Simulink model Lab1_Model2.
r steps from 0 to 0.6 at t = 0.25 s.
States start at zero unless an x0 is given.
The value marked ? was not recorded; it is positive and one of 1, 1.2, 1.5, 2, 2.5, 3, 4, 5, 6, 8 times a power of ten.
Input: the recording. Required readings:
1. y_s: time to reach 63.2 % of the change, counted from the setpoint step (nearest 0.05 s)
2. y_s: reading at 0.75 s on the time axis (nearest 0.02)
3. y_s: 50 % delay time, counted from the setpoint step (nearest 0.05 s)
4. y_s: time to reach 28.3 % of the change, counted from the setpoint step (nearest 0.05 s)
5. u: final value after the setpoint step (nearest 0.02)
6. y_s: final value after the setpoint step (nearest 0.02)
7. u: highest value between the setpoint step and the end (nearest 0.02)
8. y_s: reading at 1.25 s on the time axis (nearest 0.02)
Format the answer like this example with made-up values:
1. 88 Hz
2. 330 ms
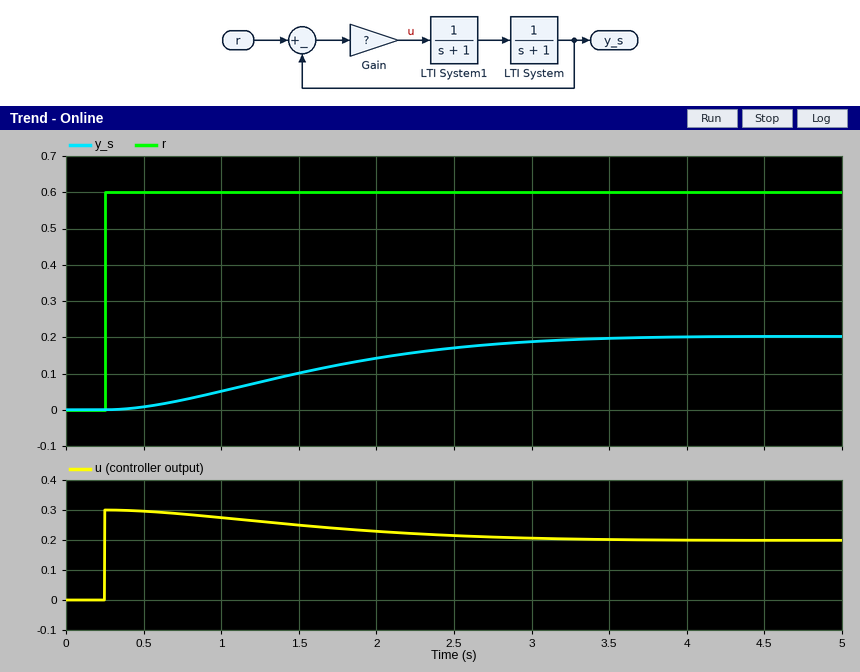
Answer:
1. 1.55 s
2. 0.02
3. 1.25 s
4. 0.80 s
5. 0.20
6. 0.20
7. 0.30
8. 0.08
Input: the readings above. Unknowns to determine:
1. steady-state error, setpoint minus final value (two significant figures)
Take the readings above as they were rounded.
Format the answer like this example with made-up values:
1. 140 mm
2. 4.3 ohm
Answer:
1. 0.40
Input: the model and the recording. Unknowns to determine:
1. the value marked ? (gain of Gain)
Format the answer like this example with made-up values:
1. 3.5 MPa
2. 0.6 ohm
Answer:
1. 0.5
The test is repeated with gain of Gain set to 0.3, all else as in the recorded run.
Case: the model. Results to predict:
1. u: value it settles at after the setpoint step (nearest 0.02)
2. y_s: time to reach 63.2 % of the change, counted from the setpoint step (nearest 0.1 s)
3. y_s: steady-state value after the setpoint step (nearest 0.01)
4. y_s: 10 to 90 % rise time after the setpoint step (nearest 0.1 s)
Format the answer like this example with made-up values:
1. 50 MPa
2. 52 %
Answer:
1. 0.14
2. 1.7 s
3. 0.14
4. 2.4 s
